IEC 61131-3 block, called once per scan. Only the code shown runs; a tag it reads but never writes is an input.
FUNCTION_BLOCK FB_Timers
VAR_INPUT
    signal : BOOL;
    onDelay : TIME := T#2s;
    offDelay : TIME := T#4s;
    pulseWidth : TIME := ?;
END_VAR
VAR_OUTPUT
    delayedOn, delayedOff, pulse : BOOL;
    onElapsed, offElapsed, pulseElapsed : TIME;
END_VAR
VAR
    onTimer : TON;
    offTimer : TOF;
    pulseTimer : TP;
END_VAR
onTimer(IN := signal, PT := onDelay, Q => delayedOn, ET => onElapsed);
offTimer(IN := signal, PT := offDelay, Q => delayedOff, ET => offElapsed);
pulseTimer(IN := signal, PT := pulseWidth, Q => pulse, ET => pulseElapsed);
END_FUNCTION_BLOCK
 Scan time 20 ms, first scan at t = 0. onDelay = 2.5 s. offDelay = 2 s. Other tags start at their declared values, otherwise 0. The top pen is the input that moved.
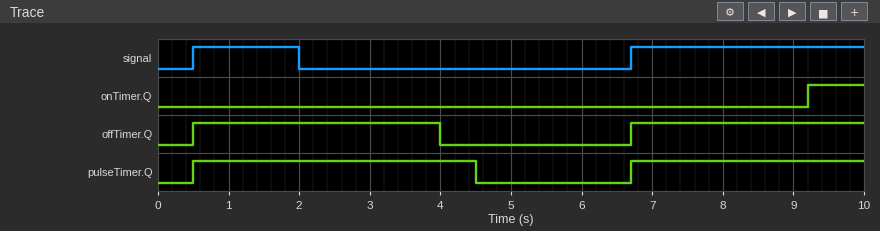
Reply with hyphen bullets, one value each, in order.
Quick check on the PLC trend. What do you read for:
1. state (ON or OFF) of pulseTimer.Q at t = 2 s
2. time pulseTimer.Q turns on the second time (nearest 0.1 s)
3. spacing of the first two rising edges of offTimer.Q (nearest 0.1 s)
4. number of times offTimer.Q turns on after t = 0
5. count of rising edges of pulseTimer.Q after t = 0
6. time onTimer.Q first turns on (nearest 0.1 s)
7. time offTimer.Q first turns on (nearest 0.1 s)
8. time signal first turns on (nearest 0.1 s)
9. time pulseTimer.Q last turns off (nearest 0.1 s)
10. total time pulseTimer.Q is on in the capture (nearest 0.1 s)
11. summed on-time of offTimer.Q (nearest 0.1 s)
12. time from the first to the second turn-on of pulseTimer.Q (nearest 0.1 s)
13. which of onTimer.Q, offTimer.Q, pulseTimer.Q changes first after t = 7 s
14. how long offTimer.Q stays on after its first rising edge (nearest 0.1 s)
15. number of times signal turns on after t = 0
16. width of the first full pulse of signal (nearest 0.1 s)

- ON
- 6.7 s
- 6.2 s
- 2
- 2
- 9.2 s
- 0.5 s
- 0.5 s
- 4.5 s
- 7.3 s
- 6.8 s
- 6.2 s
- onTimer.Q
- 3.5 s
- 2
- 1.5 s
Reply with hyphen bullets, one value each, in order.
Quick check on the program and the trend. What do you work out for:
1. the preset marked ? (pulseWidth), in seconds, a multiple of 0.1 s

- 4.0 s
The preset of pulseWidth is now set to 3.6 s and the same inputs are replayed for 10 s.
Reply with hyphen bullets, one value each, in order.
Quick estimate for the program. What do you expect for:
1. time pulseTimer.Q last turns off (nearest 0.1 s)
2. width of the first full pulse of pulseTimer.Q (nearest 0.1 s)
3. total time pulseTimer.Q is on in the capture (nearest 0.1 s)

- 4.1 s
- 3.6 s
- 6.9 s
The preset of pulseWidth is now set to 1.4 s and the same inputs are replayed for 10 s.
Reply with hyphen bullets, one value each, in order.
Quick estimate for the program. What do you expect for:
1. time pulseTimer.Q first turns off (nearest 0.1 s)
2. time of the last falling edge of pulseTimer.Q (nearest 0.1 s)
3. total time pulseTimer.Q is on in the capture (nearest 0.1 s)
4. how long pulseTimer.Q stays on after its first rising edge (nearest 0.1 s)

- 1.9 s
- 8.1 s
- 2.8 s
- 1.4 s
